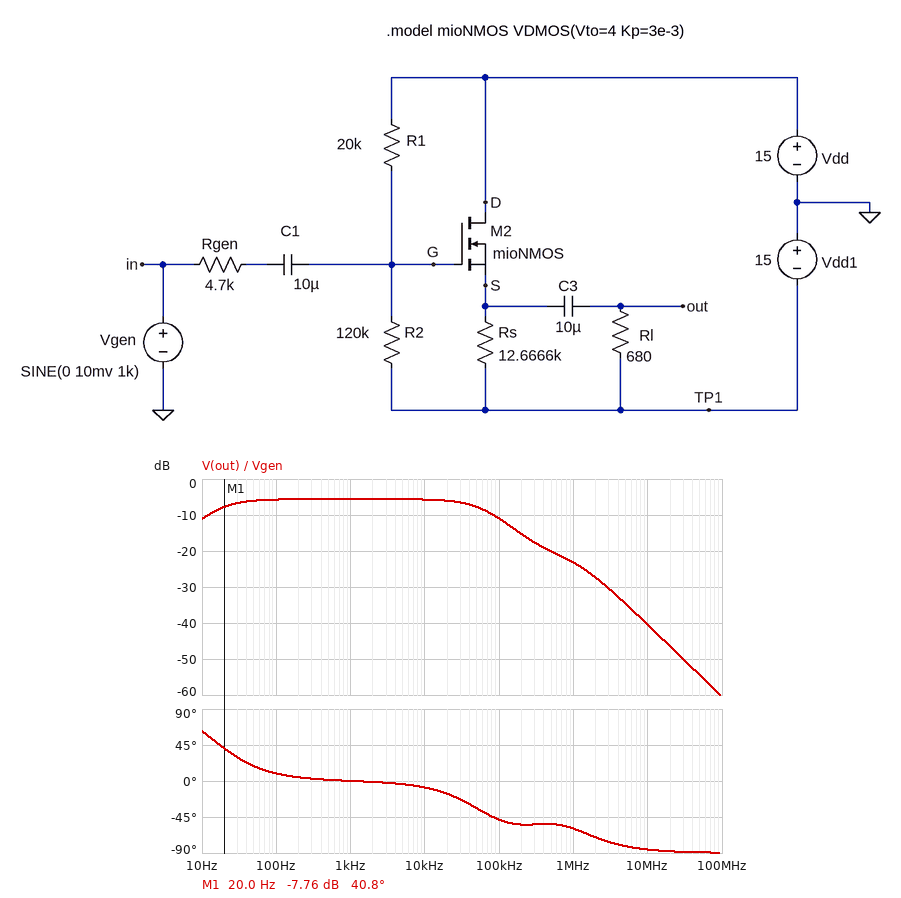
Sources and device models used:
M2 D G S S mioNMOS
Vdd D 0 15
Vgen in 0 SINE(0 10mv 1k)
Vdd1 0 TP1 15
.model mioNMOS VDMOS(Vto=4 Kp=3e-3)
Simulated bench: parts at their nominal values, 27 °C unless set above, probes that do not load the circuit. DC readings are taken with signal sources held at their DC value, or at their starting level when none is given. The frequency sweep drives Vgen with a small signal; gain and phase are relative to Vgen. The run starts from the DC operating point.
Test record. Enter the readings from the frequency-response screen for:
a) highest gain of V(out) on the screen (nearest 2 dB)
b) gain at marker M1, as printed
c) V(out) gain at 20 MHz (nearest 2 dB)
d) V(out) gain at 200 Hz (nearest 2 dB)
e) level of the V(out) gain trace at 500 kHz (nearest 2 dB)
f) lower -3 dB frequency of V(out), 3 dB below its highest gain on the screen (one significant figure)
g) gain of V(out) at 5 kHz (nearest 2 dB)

-6 dB
-7.76 dB
-46 dB
-6 dB
-20 dB
20 Hz
-6 dB
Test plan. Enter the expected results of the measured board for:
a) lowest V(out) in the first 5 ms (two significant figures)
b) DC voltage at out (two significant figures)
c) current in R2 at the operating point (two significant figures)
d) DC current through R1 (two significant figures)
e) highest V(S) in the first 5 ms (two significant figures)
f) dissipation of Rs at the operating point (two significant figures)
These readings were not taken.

-15 V
-15 V
210 µA
210 µA
5.7 V
34 mW
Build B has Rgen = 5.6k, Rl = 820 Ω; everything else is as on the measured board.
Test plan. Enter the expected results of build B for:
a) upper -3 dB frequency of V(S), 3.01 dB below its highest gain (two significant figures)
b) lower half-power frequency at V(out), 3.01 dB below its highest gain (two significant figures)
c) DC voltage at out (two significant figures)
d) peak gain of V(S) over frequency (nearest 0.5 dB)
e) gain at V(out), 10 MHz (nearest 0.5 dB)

21 kHz
14 Hz
-15 V
-3.0 dB
-42.0 dB
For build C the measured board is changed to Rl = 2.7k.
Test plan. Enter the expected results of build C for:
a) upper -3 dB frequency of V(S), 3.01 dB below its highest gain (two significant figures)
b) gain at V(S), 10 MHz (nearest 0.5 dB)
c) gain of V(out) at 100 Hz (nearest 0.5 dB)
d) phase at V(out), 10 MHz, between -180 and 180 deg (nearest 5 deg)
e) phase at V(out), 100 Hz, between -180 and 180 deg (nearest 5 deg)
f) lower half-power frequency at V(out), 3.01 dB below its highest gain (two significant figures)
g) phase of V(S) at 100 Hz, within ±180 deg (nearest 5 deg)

100 kHz
-40.5 dB
-3.5 dB
-90 deg
5 deg
5.4 Hz
0 deg
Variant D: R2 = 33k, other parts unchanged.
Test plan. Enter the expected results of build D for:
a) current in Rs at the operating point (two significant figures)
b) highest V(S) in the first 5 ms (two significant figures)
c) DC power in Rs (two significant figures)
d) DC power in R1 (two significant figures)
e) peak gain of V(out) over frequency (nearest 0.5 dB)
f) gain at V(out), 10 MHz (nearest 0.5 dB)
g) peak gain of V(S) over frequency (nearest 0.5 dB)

1.1 mA
-1.2 V
15 mW
6.4 mW
-7.0 dB
-35.5 dB
-3.5 dB
